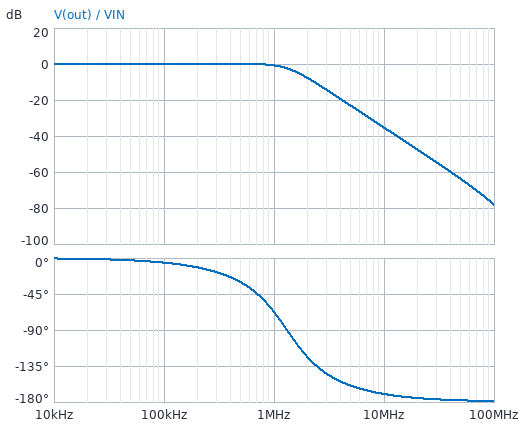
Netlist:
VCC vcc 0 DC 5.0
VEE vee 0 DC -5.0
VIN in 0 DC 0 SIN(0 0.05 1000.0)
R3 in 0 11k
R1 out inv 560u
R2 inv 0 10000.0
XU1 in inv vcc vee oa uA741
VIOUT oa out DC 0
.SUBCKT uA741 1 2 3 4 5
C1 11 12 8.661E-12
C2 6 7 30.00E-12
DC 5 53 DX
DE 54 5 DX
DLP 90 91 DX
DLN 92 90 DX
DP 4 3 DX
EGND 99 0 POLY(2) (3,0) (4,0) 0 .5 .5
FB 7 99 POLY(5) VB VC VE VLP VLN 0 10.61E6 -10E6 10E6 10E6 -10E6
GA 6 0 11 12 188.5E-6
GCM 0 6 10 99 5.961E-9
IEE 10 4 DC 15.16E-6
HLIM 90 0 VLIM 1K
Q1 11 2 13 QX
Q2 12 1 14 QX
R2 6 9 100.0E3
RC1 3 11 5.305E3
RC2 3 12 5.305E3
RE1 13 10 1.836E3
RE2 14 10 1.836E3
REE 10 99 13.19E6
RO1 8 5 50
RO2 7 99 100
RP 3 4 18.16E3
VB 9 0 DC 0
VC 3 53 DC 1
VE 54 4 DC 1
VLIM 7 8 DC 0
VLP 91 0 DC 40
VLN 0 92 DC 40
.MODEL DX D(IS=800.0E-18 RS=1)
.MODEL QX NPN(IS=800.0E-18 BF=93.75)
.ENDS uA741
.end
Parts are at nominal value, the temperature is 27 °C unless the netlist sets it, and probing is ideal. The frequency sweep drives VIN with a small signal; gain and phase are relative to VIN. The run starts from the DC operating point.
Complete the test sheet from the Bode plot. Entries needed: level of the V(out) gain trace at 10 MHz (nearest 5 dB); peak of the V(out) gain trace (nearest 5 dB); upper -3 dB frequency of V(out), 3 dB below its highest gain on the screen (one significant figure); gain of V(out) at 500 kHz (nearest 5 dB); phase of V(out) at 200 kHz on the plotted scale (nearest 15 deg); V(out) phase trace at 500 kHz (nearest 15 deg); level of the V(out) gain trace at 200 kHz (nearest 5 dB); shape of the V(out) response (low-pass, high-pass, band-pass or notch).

-35 dB
0 dB
1 MHz
0 dB
-15 deg
-30 deg
0 dB
low-pass
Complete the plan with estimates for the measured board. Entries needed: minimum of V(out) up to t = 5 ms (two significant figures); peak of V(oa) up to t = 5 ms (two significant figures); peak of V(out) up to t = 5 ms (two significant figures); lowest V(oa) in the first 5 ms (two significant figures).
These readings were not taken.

-50 mV
50 mV
50 mV
-50 mV
